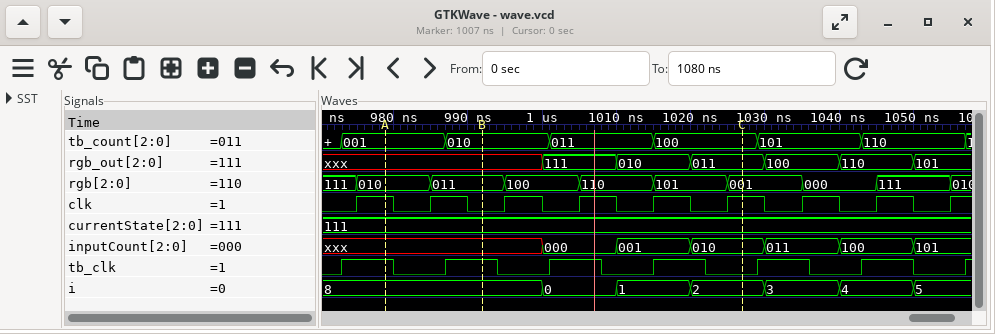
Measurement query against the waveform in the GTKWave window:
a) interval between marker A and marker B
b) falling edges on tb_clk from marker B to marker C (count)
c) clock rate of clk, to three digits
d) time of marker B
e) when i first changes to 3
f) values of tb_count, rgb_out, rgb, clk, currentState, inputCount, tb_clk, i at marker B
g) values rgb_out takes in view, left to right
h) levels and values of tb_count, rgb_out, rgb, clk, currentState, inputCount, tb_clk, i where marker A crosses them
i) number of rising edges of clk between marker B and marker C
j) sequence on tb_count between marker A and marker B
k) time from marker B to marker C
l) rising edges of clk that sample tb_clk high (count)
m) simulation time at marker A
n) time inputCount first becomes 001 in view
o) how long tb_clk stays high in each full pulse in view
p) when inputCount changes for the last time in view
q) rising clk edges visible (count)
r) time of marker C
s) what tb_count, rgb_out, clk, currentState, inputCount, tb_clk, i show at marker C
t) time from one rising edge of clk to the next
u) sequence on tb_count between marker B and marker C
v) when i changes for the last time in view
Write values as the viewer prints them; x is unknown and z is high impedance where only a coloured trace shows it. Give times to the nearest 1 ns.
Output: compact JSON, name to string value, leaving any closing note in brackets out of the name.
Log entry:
{"interval between marker A and marker B": "13 ns", "falling edges on tb_clk from marker B to marker C": "3", "clock rate of clk, to three digits": "100 MHz", "time of marker B": "992 ns", "when i first changes to 3": "1030 ns", "values of tb_count, rgb_out, rgb, clk, currentState, inputCount, tb_clk, i at marker B": "tb_count=010, rgb_out=xxx, rgb=011, clk=0, currentState=111, inputCount=xxx, tb_clk=1, i=8", "values rgb_out takes in view, left to right": "xxx, 111, 010, 011, 100, 110, 101", "levels and values of tb_count, rgb_out, rgb, clk, currentState, inputCount, tb_clk, i where marker A crosses them": "tb_count=001, rgb_out=xxx, rgb=010, clk=1, currentState=111, inputCount=xxx, tb_clk=1, i=8", "number of rising edges of clk between marker B and marker C": "4", "sequence on tb_count between marker A and marker B": "001, 010", "time from marker B to marker C": "35 ns", "rising edges of clk that sample tb_clk high": "4", "simulation time at marker A": "979 ns", "time inputCount first becomes 001 in view": "1010 ns", "how long tb_clk stays high in each full pulse in view": "7 ns, 7 ns, 7 ns, 7 ns, 7 ns, 7 ns", "when inputCount changes for the last time in view": "1050 ns", "rising clk edges visible": "9", "time of marker C": "1027 ns", "what tb_count, rgb_out, clk, currentState, inputCount, tb_clk, i show at marker C": "tb_count=100, rgb_out=011, clk=1, currentState=111, inputCount=010, tb_clk=0, i=2", "time from one rising edge of clk to the next": "10 ns", "sequence on tb_count between marker B and marker C": "010, 011, 100", "when i changes for the last time in view": "1050 ns"}
